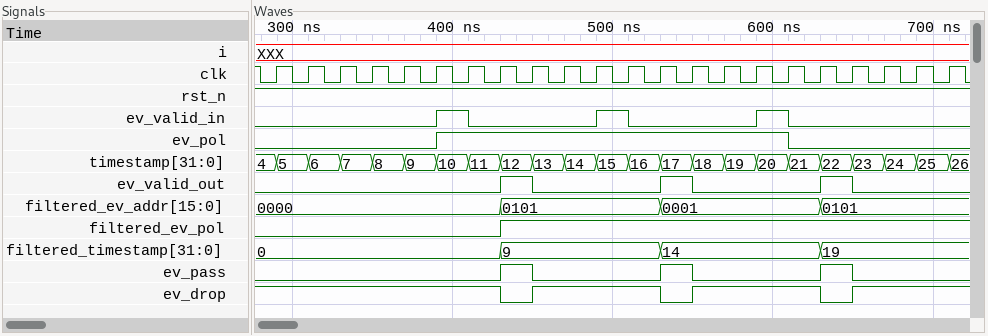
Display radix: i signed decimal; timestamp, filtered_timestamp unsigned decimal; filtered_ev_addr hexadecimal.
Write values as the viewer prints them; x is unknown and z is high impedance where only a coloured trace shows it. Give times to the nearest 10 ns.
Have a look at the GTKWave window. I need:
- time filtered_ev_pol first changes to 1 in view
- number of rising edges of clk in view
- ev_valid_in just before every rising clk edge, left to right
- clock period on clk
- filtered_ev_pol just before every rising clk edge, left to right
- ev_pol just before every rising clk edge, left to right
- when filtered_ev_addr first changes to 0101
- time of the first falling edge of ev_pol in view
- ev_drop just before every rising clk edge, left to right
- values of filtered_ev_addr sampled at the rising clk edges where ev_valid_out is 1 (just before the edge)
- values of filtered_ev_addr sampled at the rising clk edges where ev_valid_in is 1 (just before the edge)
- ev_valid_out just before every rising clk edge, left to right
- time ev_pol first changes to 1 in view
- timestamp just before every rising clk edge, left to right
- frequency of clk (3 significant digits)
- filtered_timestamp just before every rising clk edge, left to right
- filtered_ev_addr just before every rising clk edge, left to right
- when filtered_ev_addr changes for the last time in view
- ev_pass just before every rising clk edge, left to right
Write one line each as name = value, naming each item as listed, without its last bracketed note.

time filtered_ev_pol first changes to 1 in view = 430 ns
number of rising edges of clk in view = 22
ev_valid_in just before every rising clk edge, left to right = 0 0 0 0 0 0 1 0 0 0 0 1 0 0 0 0 1 0 0 0 0 0
clock period on clk = 20 ns
filtered_ev_pol just before every rising clk edge, left to right = 0 0 0 0 0 0 0 0 1 1 1 1 1 1 1 1 1 1 1 1 1 1
ev_pol just before every rising clk edge, left to right = 0 0 0 0 0 0 1 1 1 1 1 1 1 1 1 1 1 0 0 0 0 0
when filtered_ev_addr first changes to 0101 = 430 ns
time of the first falling edge of ev_pol in view = 610 ns
ev_drop just before every rising clk edge, left to right = 1 1 1 1 1 1 1 1 0 1 1 1 1 0 1 1 1 1 0 1 1 1
values of filtered_ev_addr sampled at the rising clk edges where ev_valid_out is 1 = 0101, 0001, 0101
values of filtered_ev_addr sampled at the rising clk edges where ev_valid_in is 1 = 0000, 0101, 0001
ev_valid_out just before every rising clk edge, left to right = 0 0 0 0 0 0 0 0 1 0 0 0 0 1 0 0 0 0 1 0 0 0
time ev_pol first changes to 1 in view = 390 ns
timestamp just before every rising clk edge, left to right = 4, 5, 6, 7, 8, 9, 10, 11, 12, 13, 14, 15, 16, 17, 18, 19, 20, 21, 22, 23, 24, 25
frequency of clk = 50.0 MHz
filtered_timestamp just before every rising clk edge, left to right = 0, 0, 0, 0, 0, 0, 0, 0, 9, 9, 9, 9, 9, 14, 14, 14, 14, 14, 19, 19, 19, 19
filtered_ev_addr just before every rising clk edge, left to right = 0000, 0000, 0000, 0000, 0000, 0000, 0000, 0000, 0101, 0101, 0101, 0101, 0101, 0001, 0001, 0001, 0001, 0001, 0101, 0101, 0101, 0101
when filtered_ev_addr changes for the last time in view = 630 ns
ev_pass just before every rising clk edge, left to right = 0 0 0 0 0 0 0 0 1 0 0 0 0 1 0 0 0 0 1 0 0 0
